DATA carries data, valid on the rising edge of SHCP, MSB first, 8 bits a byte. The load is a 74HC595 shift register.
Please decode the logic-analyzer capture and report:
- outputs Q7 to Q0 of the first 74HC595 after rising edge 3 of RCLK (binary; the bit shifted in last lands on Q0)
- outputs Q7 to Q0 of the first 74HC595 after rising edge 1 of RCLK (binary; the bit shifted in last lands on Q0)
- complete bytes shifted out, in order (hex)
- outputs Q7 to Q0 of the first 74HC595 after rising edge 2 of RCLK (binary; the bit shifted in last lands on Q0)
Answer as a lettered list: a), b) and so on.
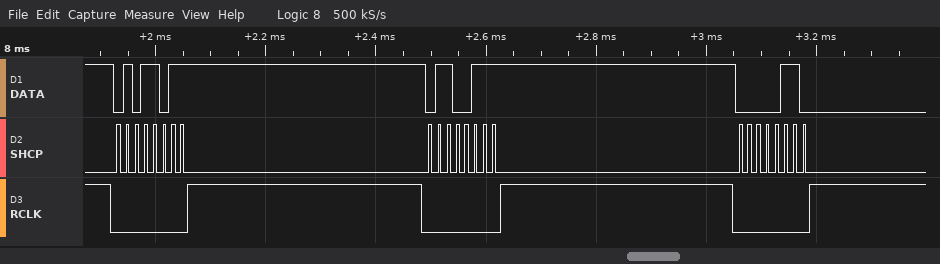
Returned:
a) 00000110
b) 01011011
c) 5B 67 06
d) 01100111
